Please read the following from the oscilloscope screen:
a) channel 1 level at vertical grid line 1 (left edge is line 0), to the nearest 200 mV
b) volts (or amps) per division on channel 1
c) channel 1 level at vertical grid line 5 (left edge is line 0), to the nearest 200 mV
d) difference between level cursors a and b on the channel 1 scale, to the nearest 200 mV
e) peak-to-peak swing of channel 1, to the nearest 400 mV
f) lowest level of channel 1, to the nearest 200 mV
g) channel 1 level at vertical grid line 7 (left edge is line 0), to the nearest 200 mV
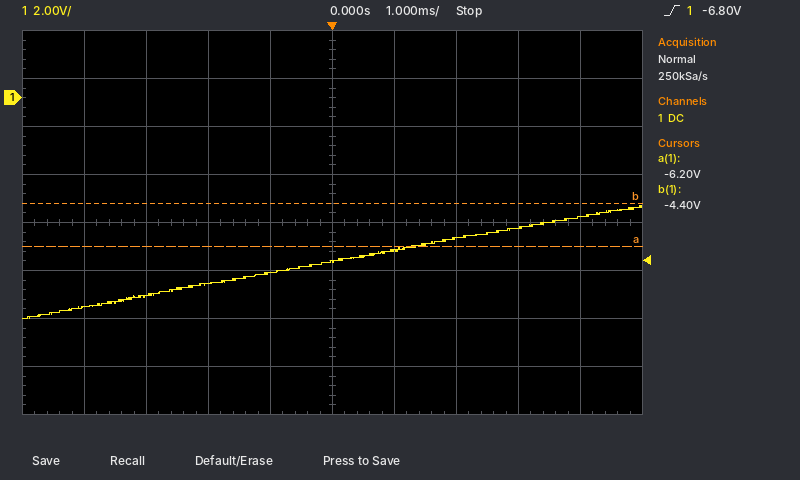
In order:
-8.8 V
2 V
-6.8 V
1.8 V
4.8 V
-9.2 V
-5.8 V
